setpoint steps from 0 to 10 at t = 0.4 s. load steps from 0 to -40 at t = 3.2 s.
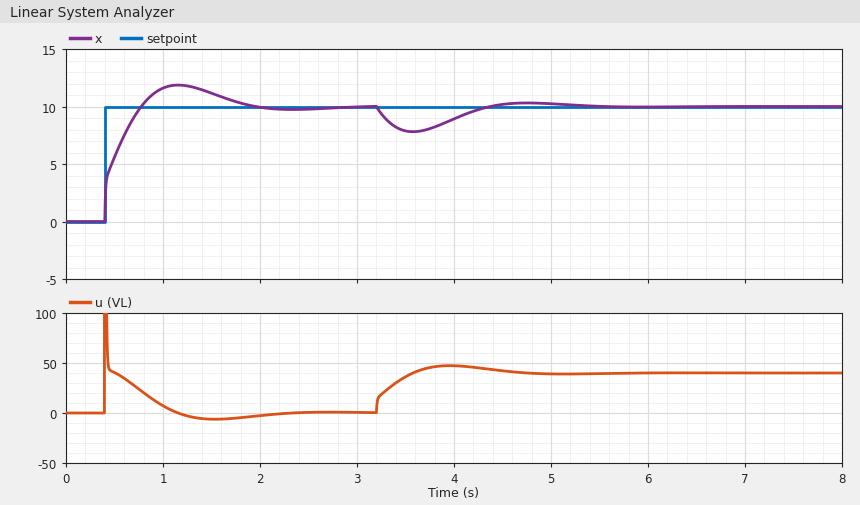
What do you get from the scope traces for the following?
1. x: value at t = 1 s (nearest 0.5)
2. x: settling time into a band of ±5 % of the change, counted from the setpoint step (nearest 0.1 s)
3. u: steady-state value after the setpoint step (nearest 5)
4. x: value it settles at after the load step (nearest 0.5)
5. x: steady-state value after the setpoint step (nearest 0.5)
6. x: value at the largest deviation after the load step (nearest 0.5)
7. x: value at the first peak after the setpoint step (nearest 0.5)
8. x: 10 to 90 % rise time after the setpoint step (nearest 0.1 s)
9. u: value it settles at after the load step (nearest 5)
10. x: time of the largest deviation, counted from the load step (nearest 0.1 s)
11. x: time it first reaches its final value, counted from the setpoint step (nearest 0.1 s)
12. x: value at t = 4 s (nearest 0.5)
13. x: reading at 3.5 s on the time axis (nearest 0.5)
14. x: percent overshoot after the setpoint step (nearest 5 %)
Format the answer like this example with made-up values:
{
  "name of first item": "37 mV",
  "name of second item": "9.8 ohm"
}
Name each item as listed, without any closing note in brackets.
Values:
{
  "x: value at t = 1 s": "11.5",
  "x: settling time into a band of ±5 % of the change, counted from the setpoint step": "1.3 s",
  "u: steady-state value after the setpoint step": "0",
  "x: value it settles at after the load step": "10.0",
  "x: steady-state value after the setpoint step": "10.0",
  "x: value at the largest deviation after the load step": "8.0",
  "x: value at the first peak after the setpoint step": "12.0",
  "x: 10 to 90 % rise time after the setpoint step": "0.3 s",
  "u: value it settles at after the load step": "40",
  "x: time of the largest deviation, counted from the load step": "0.4 s",
  "x: time it first reaches its final value, counted from the setpoint step": "0.4 s",
  "x: value at t = 4 s": "9.0",
  "x: reading at 3.5 s on the time axis": "8.0",
  "x: percent overshoot after the setpoint step": "20 %"
}
